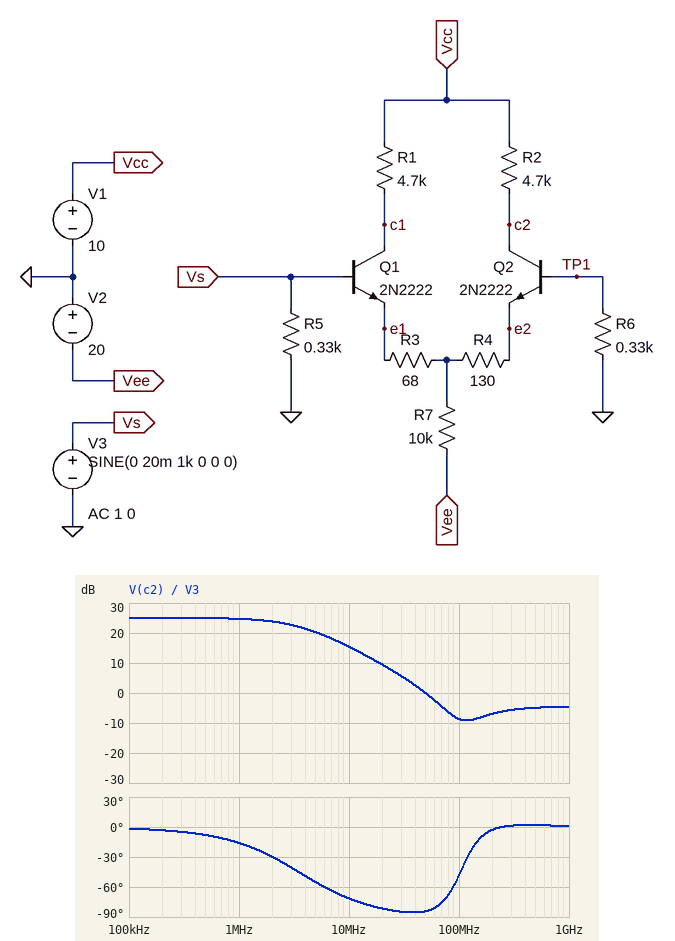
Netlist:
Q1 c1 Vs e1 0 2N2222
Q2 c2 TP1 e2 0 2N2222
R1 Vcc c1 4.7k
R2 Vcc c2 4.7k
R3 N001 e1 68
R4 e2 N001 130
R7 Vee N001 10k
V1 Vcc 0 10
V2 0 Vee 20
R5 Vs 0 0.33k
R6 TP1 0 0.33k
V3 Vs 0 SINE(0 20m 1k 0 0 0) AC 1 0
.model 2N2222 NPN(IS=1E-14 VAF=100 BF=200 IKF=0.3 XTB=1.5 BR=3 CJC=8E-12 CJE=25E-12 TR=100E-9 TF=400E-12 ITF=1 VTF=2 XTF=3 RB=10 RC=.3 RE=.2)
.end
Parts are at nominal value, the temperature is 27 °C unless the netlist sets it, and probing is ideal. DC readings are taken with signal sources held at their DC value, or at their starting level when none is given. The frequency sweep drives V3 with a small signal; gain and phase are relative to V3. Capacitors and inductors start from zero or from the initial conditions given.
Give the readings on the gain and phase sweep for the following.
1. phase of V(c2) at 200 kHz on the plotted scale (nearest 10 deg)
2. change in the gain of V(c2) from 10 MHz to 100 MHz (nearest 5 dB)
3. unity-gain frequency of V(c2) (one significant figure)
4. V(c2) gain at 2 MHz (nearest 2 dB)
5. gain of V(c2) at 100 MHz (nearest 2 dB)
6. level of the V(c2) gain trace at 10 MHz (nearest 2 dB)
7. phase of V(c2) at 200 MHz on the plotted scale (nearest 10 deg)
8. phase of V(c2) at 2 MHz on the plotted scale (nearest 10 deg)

0 deg
-25 dB
50 MHz
24 dB
-8 dB
16 dB
0 deg
-30 deg
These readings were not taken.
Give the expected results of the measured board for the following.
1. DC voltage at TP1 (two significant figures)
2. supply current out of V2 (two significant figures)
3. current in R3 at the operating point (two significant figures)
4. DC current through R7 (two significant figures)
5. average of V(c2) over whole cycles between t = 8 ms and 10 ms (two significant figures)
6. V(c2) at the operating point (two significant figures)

-1.1 mV
1.9 mA
1.2 mA
1.9 mA
6.6 V
6.6 V
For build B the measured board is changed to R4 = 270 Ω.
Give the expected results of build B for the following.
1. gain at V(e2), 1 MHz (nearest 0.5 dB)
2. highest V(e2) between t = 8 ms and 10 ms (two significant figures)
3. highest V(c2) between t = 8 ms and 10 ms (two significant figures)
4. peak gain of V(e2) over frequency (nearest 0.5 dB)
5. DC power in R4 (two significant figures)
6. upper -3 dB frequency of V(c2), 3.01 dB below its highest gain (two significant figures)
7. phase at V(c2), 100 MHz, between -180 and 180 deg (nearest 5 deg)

-15.0 dB
-630 mV
8.0 V
-6.0 dB
61 µW
4.6 MHz
-35 deg
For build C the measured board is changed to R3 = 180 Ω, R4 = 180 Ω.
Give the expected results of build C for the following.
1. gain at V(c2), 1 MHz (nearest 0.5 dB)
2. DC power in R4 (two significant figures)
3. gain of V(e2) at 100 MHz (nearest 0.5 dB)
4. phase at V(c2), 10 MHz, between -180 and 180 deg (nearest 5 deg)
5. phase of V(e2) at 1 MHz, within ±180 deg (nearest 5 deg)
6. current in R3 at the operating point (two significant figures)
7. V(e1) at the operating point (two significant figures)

20.5 dB
160 µW
-6.5 dB
-65 deg
45 deg
960 µA
-650 mV
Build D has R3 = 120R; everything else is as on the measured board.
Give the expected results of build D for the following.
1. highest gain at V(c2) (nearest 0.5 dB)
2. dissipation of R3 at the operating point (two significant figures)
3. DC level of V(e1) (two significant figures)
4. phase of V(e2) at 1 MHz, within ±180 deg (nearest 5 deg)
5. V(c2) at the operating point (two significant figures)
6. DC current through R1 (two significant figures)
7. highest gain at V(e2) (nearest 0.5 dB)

23.5 dB
120 µW
-650 mV
40 deg
5.7 V
990 µA
-5.0 dB
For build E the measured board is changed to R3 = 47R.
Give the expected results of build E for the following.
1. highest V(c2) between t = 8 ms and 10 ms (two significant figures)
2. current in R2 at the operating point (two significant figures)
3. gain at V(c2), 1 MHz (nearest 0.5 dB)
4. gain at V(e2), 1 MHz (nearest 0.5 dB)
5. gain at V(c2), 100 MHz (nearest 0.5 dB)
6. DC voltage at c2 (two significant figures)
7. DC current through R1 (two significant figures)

7.5 V
620 µA
25.5 dB
-12.0 dB
-9.0 dB
7.1 V
1.3 mA
